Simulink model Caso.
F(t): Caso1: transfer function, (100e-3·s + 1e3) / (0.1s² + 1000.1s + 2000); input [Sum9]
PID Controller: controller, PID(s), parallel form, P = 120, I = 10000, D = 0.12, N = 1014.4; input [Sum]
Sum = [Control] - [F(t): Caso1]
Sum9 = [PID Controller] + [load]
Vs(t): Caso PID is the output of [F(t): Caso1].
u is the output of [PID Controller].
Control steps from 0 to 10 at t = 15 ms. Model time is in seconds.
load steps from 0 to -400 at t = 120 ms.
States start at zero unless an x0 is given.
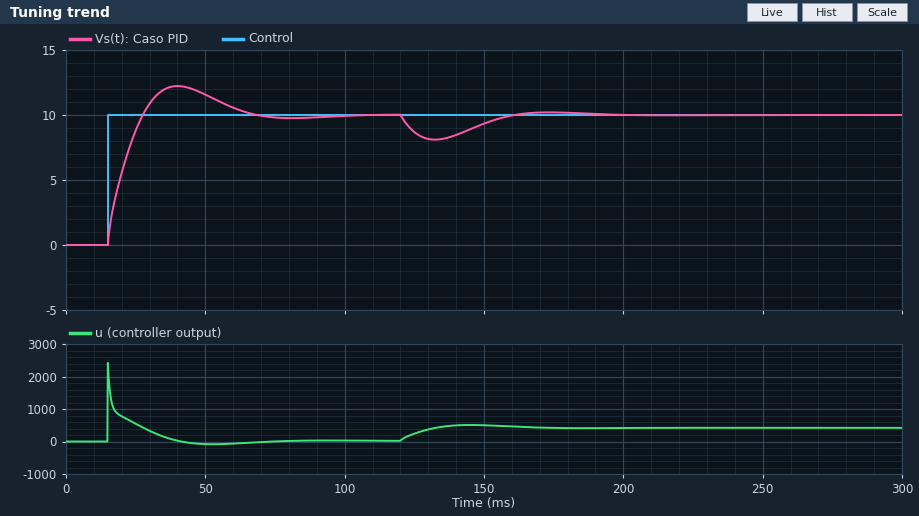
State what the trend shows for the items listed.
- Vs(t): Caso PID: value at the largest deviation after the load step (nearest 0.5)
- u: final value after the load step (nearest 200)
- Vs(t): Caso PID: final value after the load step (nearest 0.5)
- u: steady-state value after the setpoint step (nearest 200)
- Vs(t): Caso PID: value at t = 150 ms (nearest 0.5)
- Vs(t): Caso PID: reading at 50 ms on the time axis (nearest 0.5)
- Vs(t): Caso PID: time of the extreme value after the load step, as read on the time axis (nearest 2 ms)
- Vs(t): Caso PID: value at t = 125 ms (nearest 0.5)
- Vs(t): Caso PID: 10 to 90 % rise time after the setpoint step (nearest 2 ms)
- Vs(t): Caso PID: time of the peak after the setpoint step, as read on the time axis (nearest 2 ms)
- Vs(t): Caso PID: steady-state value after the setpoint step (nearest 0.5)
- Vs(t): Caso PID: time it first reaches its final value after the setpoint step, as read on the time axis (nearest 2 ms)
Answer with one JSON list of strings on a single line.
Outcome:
["8.0", "400", "10.0", "0", "9.5", "11.5", "132 ms", "8.5", "10 ms", "40 ms", "10.0", "28 ms"]
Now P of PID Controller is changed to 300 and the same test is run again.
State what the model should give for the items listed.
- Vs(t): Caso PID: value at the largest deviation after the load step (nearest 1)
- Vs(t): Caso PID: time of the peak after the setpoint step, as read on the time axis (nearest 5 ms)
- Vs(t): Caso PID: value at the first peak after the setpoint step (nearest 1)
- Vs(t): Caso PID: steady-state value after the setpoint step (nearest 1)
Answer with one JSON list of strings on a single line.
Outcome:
["9", "35 ms", "11", "10"]
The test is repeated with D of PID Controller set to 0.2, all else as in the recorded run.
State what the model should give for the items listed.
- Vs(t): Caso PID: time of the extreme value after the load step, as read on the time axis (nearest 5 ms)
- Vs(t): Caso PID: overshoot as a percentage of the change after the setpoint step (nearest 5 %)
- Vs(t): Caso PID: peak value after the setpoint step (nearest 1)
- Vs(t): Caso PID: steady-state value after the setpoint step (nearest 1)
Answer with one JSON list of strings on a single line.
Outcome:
["135 ms", "20 %", "12", "10"]
